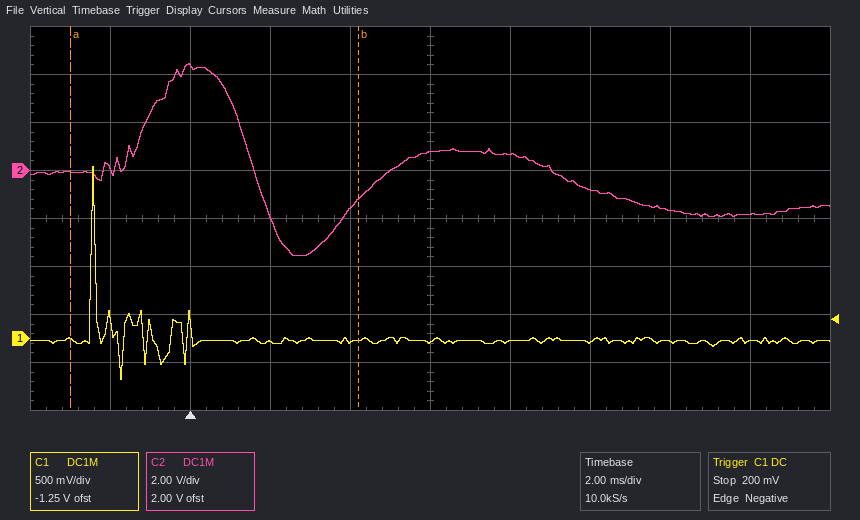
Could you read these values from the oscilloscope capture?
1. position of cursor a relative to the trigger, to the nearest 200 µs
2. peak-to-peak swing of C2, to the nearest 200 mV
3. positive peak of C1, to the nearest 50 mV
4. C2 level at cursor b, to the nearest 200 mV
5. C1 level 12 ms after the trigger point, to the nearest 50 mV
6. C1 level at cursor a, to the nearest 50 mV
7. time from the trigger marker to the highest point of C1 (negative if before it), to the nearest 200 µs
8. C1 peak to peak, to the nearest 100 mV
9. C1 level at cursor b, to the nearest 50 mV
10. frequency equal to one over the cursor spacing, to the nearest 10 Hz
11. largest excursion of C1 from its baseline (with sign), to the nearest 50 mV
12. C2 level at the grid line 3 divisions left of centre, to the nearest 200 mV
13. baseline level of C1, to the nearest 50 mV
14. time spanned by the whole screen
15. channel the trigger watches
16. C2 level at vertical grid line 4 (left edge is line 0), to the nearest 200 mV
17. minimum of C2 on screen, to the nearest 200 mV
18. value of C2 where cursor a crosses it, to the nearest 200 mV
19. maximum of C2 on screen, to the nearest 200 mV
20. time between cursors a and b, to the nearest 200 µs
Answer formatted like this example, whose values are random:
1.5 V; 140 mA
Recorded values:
-3.0 ms; 8.0 V; 1.80 V; -1.2 V; -50 mV; 0 mV; -2.4 ms; 2.20 V; 0 mV; 140 Hz; +1.80 V; 4.4 V; 0 mV; 20 ms; C1; -1.6 V; -3.6 V; 0.0 V; 4.4 V; 7.2 ms
